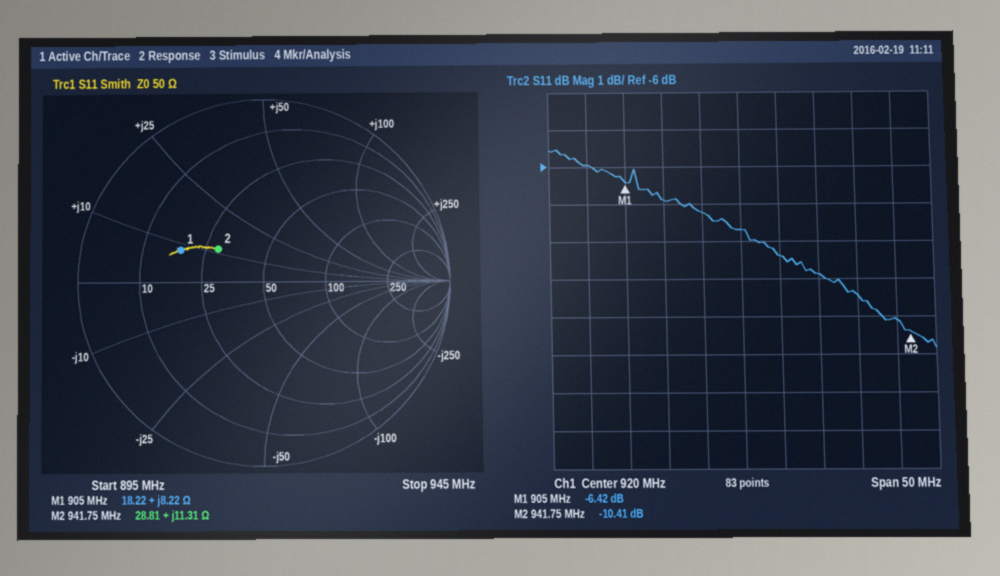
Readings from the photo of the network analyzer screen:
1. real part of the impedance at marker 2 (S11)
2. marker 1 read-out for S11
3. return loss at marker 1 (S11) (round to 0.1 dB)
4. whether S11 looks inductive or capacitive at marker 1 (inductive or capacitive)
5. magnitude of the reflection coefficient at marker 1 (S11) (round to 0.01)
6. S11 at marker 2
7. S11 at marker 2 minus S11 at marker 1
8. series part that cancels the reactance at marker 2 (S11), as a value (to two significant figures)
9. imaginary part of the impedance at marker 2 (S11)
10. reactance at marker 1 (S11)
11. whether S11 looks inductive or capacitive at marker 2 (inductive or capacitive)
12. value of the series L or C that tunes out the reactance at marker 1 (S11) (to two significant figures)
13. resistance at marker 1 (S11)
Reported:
28.81 Ω
-6.42 dB
6.4 dB
inductive
0.48
-10.41 dB
-3.99 dB
15 pF
+11.31 Ω
+8.22 Ω
inductive
21 pF
18.22 Ω
